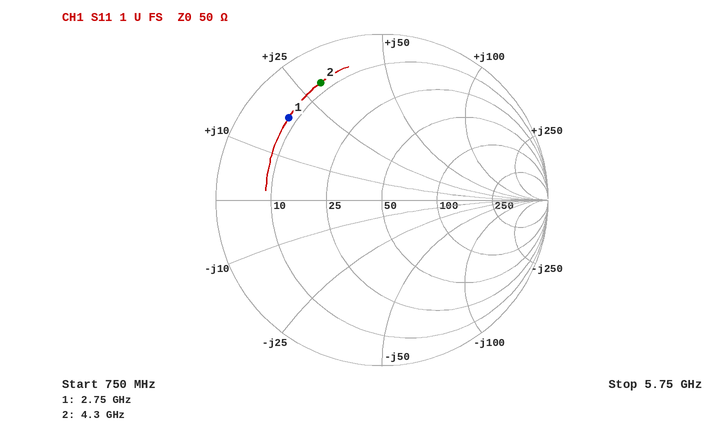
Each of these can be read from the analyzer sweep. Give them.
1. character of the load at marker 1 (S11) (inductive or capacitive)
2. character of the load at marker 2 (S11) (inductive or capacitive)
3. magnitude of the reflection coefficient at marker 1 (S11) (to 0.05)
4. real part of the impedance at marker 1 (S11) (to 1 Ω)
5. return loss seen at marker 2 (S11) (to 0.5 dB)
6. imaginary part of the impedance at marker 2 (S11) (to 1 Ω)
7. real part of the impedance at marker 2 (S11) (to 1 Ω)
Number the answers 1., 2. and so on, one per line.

1. inductive
2. inductive
3. 0.75
4. 8 Ω
5. 2.0 dB
6. +30 Ω
7. 8 Ω
